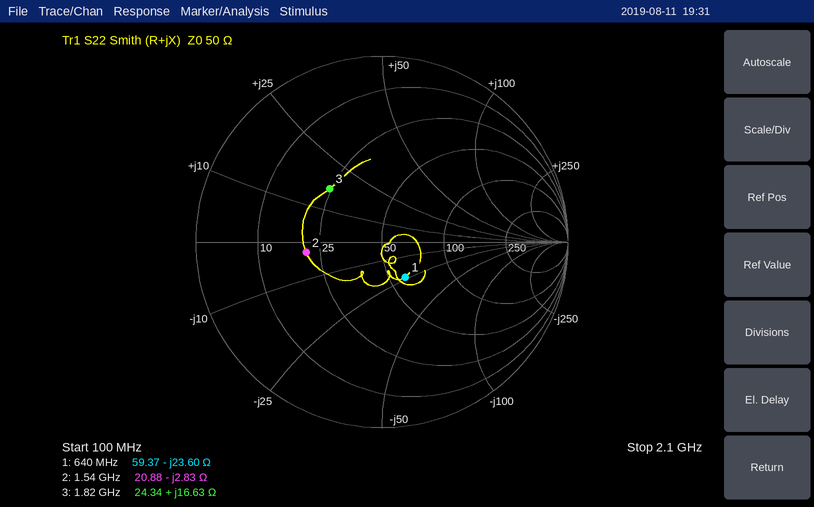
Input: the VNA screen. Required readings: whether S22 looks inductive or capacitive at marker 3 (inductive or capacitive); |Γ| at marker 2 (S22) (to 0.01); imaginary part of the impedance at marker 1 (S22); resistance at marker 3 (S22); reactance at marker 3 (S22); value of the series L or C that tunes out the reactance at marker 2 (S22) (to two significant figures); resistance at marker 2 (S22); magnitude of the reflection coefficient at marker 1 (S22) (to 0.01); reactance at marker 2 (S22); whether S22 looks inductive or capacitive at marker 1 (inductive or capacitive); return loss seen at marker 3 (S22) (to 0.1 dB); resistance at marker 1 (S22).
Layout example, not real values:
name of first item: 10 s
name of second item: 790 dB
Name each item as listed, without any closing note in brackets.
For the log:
whether S22 looks inductive or capacitive at marker 3: inductive
|Γ| at marker 2 (S22): 0.41
imaginary part of the impedance at marker 1: -23.60 Ω
resistance at marker 3: 24.34 Ω
reactance at marker 3: +16.63 Ω
value of the series L or C that tunes out the reactance at marker 2 (S22): 290 pH
resistance at marker 2: 20.88 Ω
magnitude of the reflection coefficient at marker 1 (S22): 0.23
reactance at marker 2: -2.83 Ω
whether S22 looks inductive or capacitive at marker 1: capacitive
return loss seen at marker 3 (S22): 7.9 dB
resistance at marker 1: 59.37 Ω
